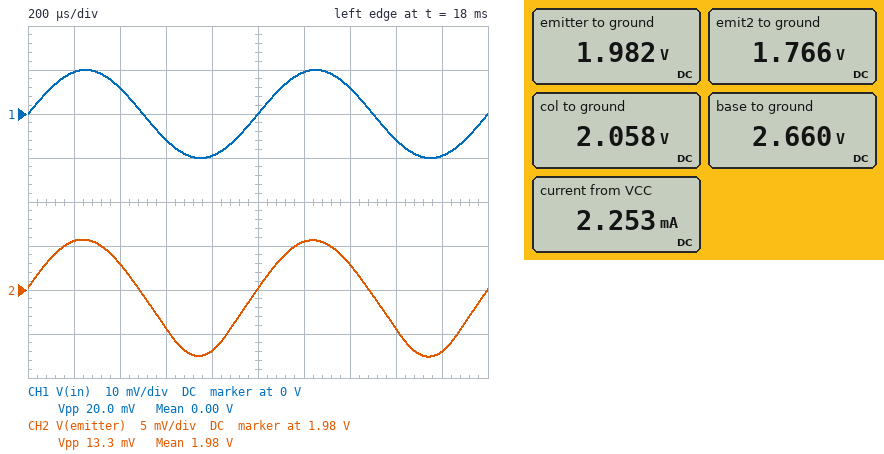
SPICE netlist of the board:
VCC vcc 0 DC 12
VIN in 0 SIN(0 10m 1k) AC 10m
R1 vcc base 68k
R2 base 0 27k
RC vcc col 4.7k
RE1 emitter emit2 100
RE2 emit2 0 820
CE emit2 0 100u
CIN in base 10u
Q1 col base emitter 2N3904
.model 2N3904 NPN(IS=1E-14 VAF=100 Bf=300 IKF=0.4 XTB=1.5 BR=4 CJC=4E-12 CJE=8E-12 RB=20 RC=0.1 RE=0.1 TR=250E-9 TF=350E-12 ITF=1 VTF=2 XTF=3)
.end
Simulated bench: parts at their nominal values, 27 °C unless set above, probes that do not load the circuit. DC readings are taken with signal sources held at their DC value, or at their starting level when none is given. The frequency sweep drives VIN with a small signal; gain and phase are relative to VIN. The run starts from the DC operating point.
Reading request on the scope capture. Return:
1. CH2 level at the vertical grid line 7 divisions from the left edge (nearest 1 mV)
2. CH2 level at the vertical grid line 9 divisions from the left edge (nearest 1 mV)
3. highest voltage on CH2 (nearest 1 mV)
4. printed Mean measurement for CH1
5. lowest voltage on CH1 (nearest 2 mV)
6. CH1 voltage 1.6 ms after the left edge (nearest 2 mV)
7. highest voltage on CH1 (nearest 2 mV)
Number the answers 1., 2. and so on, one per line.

1. 1.983 V
2. 1.973 V
3. 1.986 V
4. 0.00 V
5. -10 mV
6. -6 mV
7. 10 mV
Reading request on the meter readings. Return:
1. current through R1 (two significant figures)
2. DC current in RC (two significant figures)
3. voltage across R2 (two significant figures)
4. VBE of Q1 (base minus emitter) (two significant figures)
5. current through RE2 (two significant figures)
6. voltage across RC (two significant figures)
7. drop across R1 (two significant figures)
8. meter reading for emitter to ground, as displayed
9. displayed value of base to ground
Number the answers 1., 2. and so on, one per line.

1. 140 µA
2. 2.1 mA
3. 2.7 V
4. 680 mV
5. 2.2 mA
6. 9.9 V
7. 9.3 V
8. 1.982 V
9. 2.660 V
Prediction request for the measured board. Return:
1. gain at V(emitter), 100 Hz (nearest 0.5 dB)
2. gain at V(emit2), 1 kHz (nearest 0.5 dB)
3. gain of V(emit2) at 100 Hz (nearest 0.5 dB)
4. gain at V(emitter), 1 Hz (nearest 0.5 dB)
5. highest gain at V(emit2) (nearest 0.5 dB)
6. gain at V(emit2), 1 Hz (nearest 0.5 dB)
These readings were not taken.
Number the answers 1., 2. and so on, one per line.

1. -7.0 dB
2. -40.5 dB
3. -23.0 dB
4. -26.5 dB
5. -20.0 dB
6. -27.5 dB
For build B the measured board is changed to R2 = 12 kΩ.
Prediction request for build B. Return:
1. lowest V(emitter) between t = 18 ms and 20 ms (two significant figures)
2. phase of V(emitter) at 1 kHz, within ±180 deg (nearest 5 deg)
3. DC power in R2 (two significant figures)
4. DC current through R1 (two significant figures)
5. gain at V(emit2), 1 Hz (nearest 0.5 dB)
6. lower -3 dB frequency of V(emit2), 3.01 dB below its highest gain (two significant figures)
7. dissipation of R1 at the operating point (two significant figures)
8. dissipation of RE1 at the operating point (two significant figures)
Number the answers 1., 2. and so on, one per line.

1. 1.1 V
2. 0 deg
3. 260 µW
4. 150 µA
5. -7.0 dB
6. 1.3 Hz
7. 1.5 mW
8. 140 µW
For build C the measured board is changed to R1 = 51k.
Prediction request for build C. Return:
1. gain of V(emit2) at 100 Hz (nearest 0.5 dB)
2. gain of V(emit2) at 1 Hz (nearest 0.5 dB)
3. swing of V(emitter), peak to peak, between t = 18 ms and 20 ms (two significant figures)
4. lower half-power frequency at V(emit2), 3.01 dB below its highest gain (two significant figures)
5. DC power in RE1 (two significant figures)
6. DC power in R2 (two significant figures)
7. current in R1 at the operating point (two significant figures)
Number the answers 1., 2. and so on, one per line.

1. -23.5 dB
2. -28.0 dB
3. 12 mV
4. 2.1 Hz
5. 480 µW
6. 270 µW
7. 180 µA
